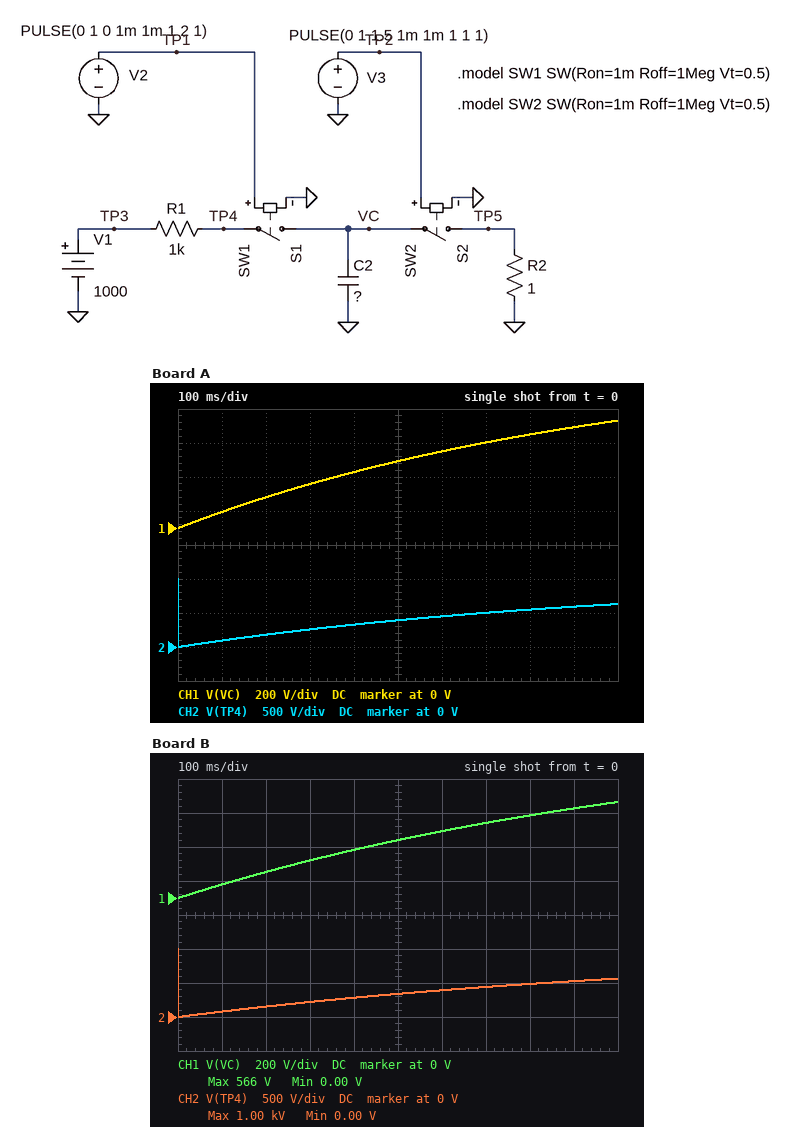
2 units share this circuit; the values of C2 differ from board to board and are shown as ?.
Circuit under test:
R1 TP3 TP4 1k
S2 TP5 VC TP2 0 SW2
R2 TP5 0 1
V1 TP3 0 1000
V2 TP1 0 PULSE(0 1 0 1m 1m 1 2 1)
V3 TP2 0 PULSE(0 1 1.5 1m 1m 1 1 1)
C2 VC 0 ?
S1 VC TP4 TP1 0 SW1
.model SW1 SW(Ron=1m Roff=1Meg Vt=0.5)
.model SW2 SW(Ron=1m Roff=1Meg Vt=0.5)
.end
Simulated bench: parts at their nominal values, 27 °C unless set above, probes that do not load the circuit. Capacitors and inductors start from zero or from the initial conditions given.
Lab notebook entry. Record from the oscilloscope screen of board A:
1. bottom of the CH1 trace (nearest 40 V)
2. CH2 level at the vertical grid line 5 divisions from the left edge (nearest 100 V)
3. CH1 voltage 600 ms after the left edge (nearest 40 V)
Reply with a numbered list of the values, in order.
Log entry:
1. 0 V
2. 400 V
3. 440 V
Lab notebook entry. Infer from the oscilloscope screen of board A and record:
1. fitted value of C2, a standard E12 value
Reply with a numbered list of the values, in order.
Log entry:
1. 1 mF
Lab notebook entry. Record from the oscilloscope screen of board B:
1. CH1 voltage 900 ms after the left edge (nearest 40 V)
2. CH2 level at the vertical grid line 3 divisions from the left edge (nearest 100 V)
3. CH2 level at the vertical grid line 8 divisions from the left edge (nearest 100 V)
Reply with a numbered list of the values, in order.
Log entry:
1. 520 V
2. 200 V
3. 500 V
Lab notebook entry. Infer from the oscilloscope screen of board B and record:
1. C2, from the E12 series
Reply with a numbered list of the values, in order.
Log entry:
1. 1.2 mF
